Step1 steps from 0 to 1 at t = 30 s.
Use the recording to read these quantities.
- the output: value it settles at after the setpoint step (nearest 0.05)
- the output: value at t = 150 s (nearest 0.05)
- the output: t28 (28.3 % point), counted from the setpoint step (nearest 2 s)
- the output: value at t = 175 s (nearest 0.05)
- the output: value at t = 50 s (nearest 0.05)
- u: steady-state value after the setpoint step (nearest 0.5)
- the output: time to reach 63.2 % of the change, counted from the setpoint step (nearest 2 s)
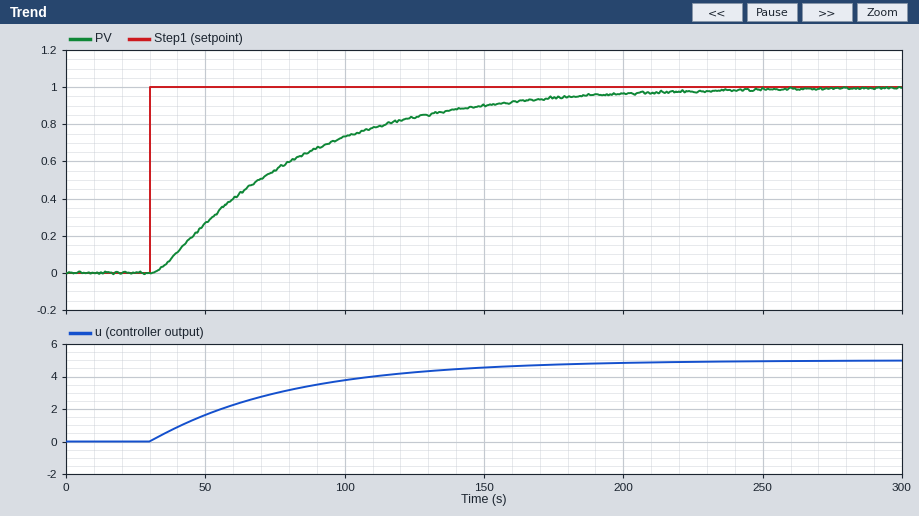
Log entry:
1.00
0.90
22 s
0.95
0.25
5.0
54 s
